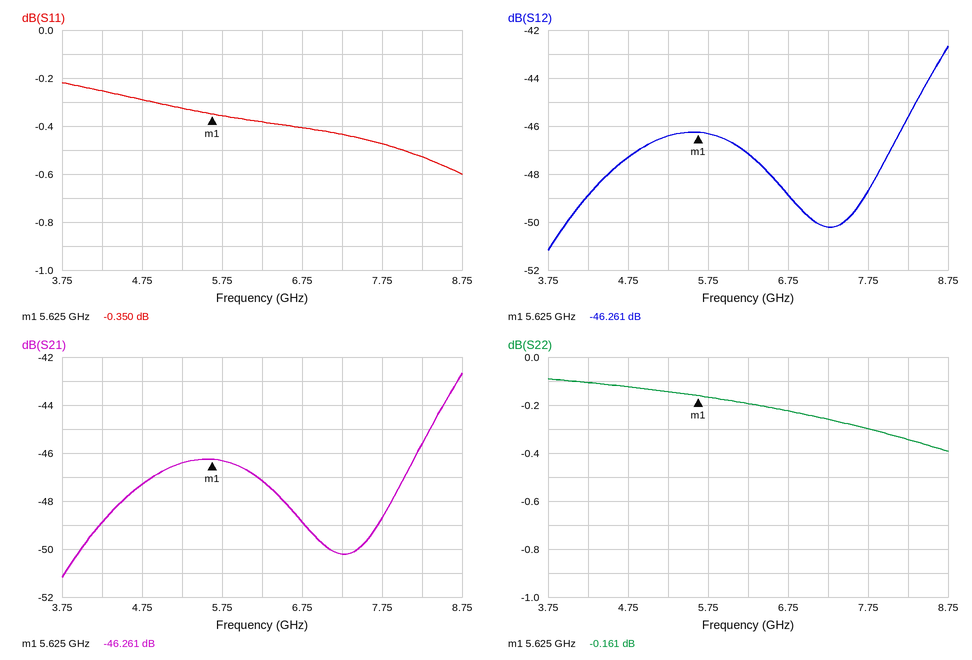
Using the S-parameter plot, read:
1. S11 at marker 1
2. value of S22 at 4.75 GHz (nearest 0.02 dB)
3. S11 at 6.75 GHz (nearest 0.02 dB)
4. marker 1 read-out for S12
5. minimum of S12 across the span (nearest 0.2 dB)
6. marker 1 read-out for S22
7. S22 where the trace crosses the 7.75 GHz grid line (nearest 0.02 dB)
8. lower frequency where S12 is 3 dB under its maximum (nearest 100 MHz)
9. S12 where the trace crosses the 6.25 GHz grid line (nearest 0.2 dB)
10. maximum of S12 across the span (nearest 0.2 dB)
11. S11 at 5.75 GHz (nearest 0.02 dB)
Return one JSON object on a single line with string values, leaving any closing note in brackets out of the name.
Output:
{"S11 at marker 1": "-0.350 dB", "value of S22 at 4.75 GHz": "-0.12 dB", "S11 at 6.75 GHz": "-0.40 dB", "marker 1 read-out for S12": "-46.261 dB", "minimum of S12 across the span": "-51.2 dB", "marker 1 read-out for S22": "-0.161 dB", "S22 where the trace crosses the 7.75 GHz grid line": "-0.30 dB", "lower frequency where S12 is 3 dB under its maximum": "8.2 GHz", "S12 where the trace crosses the 6.25 GHz grid line": "-47.2 dB", "maximum of S12 across the span": "-42.6 dB", "S11 at 5.75 GHz": "-0.36 dB"}
